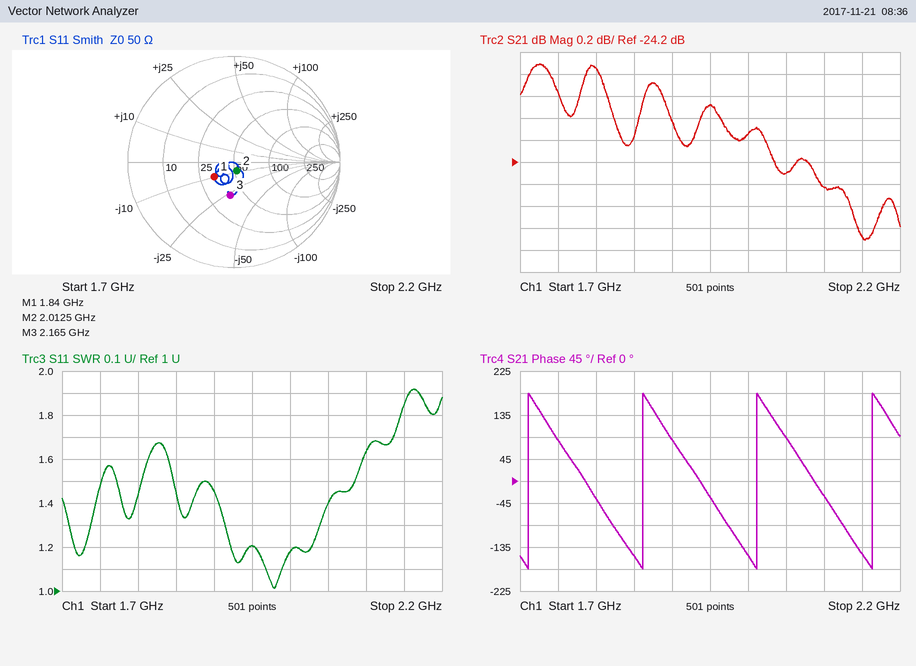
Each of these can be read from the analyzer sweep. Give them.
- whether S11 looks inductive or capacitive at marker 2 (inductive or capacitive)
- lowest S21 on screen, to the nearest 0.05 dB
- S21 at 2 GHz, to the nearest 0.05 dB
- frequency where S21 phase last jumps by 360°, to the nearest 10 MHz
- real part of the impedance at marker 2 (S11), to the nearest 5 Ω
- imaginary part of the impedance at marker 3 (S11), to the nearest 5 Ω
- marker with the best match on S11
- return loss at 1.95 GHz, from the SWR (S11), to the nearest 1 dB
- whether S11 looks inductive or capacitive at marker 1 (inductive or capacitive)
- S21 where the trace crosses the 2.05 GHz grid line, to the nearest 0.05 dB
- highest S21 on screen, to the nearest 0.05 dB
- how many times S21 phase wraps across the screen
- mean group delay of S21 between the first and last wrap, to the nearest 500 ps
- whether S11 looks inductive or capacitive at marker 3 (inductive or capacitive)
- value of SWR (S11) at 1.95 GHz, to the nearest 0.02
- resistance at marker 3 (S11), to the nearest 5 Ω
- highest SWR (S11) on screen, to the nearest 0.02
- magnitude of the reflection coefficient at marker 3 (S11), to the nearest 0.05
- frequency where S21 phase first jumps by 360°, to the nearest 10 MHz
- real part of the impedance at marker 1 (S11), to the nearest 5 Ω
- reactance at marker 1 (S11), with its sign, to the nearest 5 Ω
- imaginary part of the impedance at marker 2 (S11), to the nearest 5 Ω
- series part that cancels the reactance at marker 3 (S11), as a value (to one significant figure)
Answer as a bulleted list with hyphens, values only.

- capacitive
- -24.90 dB
- -23.95 dB
- 2.16 GHz
- 50 Ω
- -25 Ω
- marker 2
- 21 dB
- capacitive
- -24.30 dB
- -23.30 dB
- 4
- 6.5 ns
- capacitive
- 1.20
- 40 Ω
- 1.92
- 0.30
- 1.71 GHz
- 35 Ω
- -10 Ω
- -10 Ω
- 2 nH
